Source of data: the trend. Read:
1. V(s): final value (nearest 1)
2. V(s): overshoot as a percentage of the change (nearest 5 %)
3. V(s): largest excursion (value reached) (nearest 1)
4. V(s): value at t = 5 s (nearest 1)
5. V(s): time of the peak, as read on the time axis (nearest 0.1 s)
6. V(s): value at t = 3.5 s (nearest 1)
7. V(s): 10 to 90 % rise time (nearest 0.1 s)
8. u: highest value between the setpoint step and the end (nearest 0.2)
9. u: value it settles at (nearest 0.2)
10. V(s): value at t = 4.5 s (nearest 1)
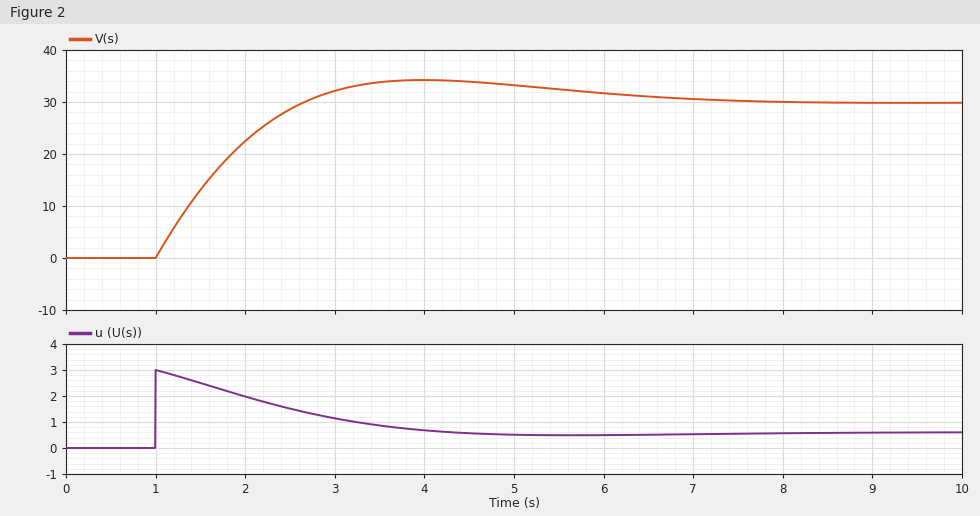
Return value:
30
15 %
34
33
4.0 s
34
1.2 s
3.0
0.6
34
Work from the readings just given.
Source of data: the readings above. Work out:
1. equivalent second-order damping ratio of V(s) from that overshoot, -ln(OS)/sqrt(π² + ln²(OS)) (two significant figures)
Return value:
0.52
